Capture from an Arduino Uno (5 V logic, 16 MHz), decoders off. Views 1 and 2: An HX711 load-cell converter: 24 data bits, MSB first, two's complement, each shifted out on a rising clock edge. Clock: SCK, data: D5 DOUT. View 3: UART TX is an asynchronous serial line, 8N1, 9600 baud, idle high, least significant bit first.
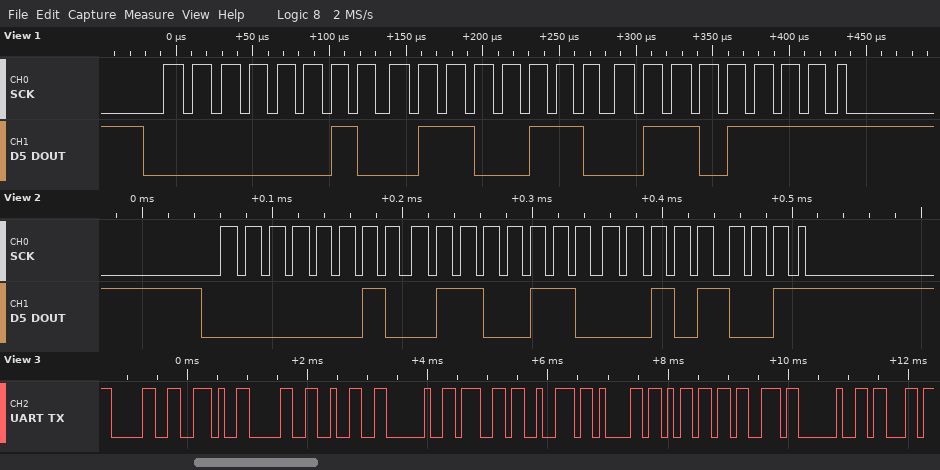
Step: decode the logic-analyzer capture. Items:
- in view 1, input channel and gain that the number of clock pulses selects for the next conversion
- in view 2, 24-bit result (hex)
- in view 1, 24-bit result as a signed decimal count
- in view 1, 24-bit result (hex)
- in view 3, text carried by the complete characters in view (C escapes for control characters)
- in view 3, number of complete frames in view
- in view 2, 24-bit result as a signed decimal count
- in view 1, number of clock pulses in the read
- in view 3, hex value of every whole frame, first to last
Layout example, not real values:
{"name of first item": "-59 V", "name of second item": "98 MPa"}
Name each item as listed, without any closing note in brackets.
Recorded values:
{"in view 1, input channel and gain that the number of clock pulses selects for the next conversion": "channel A, gain 128", "in view 2, 24-bit result": "0x026629", "in view 1, 24-bit result as a signed decimal count": "157295", "in view 1, 24-bit result": "0x02666F", "in view 3, text carried by the complete characters in view": "\"0.02 grams c\"", "in view 3, number of complete frames in view": "12", "in view 2, 24-bit result as a signed decimal count": "157225", "in view 1, number of clock pulses in the read": "25", "in view 3, hex value of every whole frame, first to last": "0x30 0x2E 0x30 0x32 0x20 0x67 0x72 0x61 0x6D 0x73 0x20 0x63"}
